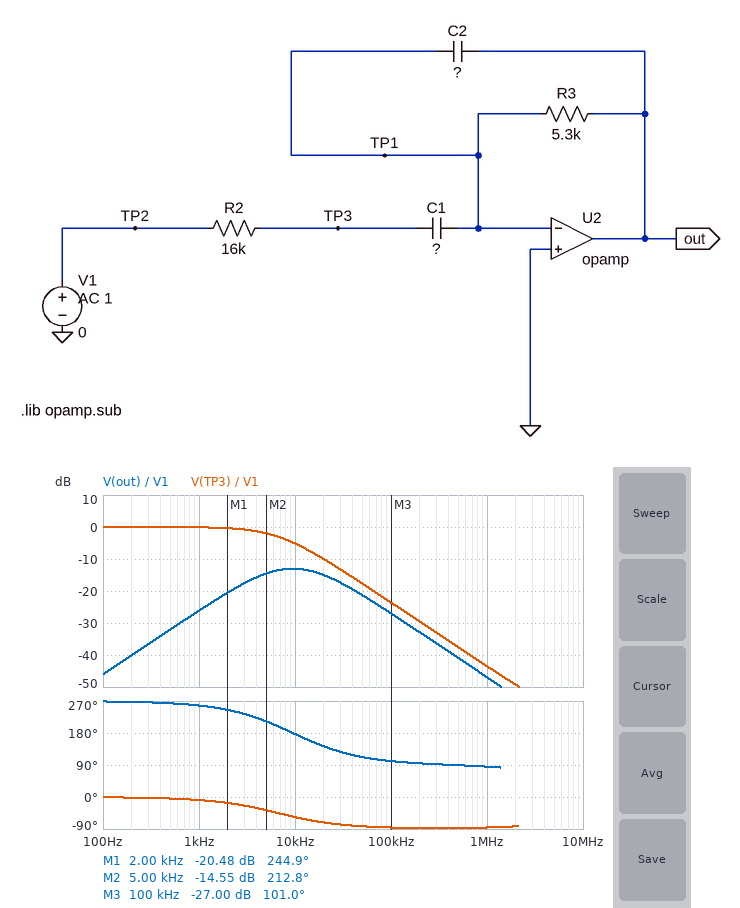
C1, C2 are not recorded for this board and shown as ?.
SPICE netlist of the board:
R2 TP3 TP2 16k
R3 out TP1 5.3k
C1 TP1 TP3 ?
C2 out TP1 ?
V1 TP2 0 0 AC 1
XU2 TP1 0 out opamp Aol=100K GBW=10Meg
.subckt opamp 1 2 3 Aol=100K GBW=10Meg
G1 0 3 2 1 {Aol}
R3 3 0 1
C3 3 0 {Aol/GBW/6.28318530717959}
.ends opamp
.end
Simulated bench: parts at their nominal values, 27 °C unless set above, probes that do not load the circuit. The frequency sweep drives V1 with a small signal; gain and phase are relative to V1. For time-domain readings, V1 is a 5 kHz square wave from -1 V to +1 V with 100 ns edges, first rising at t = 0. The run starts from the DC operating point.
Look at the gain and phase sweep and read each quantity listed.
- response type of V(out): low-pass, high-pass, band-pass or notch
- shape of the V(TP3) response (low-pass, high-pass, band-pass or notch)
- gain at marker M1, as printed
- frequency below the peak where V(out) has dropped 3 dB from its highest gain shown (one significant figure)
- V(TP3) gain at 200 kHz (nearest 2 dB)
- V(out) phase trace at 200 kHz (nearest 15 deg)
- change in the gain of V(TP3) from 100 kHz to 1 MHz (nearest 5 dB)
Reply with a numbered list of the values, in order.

1. band-pass
2. low-pass
3. -20.48 dB
4. 4 kHz
5. -30 dB
6. 90 deg
7. -20 dB
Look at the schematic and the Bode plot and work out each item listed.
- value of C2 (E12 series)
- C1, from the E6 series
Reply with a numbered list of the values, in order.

1. 2.2 nF
2. 1.5 nF
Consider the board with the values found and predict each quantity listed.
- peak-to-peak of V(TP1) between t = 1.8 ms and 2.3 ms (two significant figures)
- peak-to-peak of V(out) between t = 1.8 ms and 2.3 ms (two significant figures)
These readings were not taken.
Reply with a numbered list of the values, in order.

1. 1.8 mV
2. 650 mV
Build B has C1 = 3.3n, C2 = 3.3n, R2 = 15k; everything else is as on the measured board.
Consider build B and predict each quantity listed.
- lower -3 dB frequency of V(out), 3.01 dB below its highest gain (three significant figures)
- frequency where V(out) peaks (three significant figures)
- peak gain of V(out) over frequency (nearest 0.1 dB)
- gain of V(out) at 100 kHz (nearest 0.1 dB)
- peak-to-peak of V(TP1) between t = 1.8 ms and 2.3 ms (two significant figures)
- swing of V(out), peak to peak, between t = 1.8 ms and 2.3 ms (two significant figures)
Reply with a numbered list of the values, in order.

1. 2.04 kHz
2. 5.41 kHz
3. -11.7 dB
4. -29.9 dB
5. 1.4 mV
6. 660 mV
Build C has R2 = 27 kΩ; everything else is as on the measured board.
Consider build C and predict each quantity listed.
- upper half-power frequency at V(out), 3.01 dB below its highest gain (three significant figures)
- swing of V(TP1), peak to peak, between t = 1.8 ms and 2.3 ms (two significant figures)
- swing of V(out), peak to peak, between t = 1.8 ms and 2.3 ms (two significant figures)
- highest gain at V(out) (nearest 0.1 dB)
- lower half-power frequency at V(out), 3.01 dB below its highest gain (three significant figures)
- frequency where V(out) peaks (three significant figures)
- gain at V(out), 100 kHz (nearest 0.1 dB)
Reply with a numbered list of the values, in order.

1. 20.2 kHz
2. 1.1 mV
3. 420 mV
4. -16.3 dB
5. 2.65 kHz
6. 7.32 kHz
7. -31.5 dB
